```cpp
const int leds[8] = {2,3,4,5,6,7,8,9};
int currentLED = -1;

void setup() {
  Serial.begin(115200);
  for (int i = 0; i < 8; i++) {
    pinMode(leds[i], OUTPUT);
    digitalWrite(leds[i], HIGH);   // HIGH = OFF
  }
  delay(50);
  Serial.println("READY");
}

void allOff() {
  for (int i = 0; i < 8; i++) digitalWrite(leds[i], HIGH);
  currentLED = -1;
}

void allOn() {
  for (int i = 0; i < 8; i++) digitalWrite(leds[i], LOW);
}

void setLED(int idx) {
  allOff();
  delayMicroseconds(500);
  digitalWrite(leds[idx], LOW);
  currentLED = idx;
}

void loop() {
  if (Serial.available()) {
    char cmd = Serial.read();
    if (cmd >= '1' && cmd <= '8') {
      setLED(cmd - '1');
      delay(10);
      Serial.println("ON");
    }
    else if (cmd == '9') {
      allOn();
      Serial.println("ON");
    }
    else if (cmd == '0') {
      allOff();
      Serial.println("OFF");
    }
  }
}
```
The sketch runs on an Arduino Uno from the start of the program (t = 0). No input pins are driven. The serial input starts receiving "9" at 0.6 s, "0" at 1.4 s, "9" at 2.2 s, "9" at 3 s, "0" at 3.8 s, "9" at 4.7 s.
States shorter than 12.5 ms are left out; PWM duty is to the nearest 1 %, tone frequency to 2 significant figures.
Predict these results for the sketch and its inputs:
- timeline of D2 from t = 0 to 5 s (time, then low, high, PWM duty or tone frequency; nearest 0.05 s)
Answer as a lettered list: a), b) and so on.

a) 0 s high; 0.6 s low; 1.4 s high; 2.2 s low; 3.8 s high; 4.7 s low
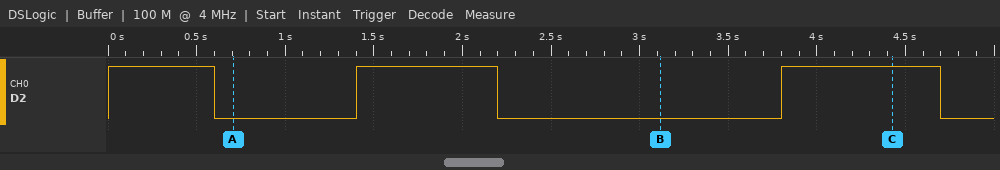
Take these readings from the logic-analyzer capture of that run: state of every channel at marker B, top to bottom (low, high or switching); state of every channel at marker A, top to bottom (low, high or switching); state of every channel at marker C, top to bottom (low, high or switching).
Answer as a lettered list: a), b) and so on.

a) D2 low
b) D2 low
c) D2 high
